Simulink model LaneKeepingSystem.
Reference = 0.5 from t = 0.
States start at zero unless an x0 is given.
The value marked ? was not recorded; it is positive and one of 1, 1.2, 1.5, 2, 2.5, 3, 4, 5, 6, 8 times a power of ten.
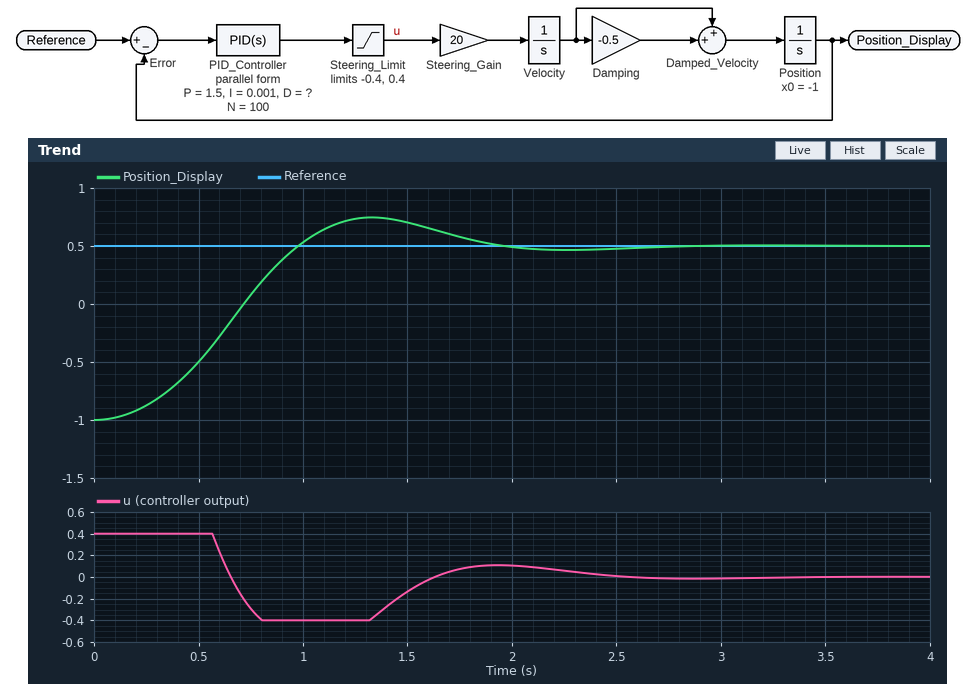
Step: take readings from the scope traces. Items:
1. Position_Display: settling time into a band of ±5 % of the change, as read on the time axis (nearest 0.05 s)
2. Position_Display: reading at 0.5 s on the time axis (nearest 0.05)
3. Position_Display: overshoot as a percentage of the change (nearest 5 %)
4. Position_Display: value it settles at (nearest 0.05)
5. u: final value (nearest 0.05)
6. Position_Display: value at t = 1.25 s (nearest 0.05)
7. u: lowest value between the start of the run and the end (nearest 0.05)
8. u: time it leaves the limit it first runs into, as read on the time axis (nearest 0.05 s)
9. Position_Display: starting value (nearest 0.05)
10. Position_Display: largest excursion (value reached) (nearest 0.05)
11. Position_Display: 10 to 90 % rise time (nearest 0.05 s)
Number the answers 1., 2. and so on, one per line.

1. 1.75 s
2. -0.50
3. 15 %
4. 0.50
5. 0.00
6. 0.75
7. -0.40
8. 0.55 s
9. -1.00
10. 0.75
11. 0.60 s
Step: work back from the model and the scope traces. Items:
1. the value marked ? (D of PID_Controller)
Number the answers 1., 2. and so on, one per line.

1. 0.4
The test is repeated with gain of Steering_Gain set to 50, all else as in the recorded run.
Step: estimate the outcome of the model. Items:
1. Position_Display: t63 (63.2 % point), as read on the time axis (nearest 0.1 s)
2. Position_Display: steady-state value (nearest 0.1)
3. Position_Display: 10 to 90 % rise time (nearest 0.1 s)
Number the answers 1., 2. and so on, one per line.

1. 0.5 s
2. 0.5
3. 0.5 s
